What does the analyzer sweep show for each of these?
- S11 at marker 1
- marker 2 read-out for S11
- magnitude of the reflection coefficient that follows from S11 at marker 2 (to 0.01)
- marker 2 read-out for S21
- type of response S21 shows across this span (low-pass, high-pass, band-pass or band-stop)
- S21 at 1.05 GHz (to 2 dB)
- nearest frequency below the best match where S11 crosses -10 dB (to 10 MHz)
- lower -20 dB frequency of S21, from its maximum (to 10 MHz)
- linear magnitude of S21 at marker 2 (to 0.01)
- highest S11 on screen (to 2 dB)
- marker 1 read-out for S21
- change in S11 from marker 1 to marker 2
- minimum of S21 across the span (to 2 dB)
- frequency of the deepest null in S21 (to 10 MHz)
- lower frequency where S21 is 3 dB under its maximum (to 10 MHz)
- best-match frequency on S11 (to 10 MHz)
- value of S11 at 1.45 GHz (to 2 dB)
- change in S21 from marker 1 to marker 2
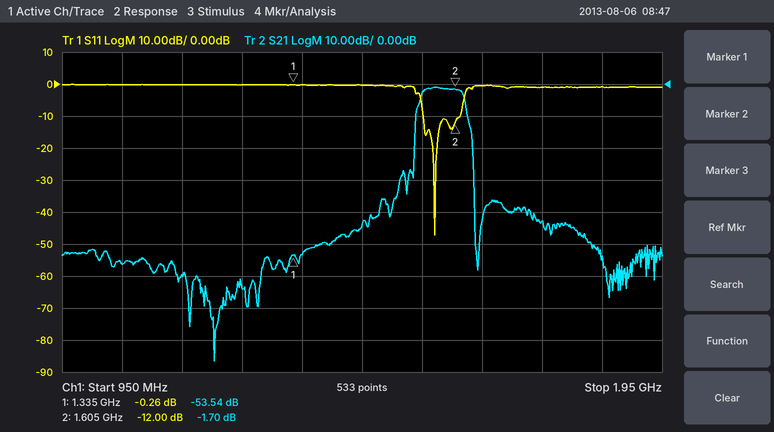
-0.26 dB
-12.00 dB
0.25
-1.70 dB
band-pass
-56 dB
1.55 GHz
1.54 GHz
0.82
0 dB
-53.54 dB
-11.74 dB
-86 dB
1.20 GHz
1.55 GHz
1.57 GHz
0 dB
51.84 dB
